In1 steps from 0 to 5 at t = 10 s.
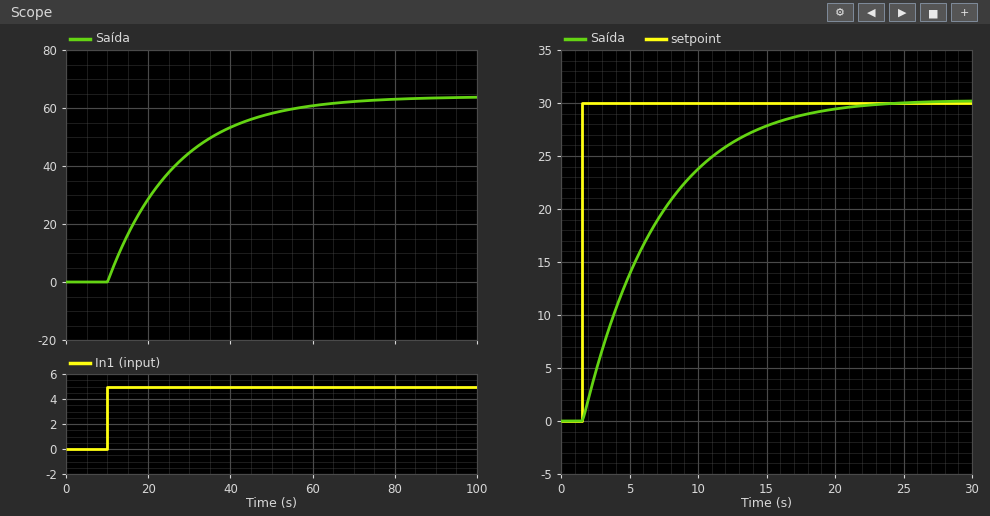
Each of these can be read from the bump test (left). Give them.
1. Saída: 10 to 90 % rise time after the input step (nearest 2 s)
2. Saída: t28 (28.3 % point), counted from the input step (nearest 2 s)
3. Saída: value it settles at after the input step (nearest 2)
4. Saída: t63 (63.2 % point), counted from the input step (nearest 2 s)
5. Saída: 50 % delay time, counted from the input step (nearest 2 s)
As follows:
36 s
6 s
64
16 s
12 s
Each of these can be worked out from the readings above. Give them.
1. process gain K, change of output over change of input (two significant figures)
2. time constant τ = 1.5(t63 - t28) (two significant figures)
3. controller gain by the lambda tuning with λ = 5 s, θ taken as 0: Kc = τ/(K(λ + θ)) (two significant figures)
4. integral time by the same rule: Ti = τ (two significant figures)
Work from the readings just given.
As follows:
13
15 s
0.23
15 s
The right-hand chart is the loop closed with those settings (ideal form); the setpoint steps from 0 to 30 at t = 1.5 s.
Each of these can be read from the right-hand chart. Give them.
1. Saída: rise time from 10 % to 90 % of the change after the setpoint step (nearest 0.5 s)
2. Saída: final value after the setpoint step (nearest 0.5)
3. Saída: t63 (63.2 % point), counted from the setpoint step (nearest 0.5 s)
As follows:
11.5 s
30.0
5.5 s
